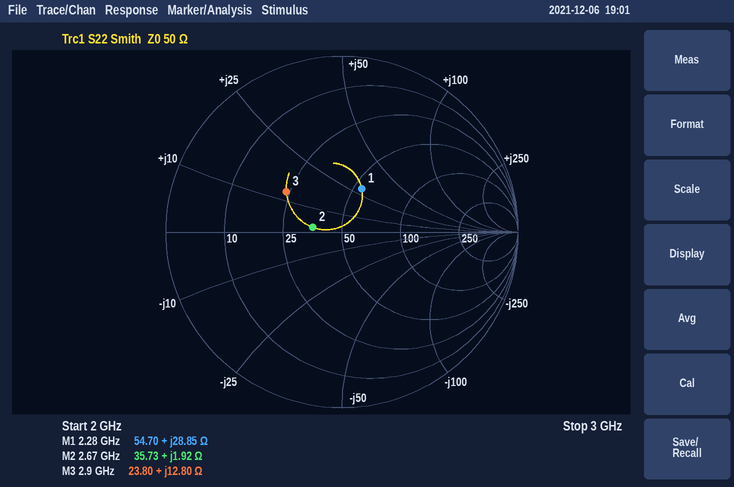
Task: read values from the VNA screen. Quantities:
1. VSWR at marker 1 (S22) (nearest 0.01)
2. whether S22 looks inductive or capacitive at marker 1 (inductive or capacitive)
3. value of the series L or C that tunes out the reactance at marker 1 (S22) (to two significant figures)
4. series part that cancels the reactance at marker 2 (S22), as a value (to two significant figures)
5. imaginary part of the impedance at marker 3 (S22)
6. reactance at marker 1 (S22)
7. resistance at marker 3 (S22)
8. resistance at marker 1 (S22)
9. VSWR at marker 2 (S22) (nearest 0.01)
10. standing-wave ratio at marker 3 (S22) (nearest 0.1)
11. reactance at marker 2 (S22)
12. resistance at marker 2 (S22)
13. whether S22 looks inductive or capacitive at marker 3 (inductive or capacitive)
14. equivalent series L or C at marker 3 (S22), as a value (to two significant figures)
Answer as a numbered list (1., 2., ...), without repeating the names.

1. 1.74
2. inductive
3. 2.4 pF
4. 31 pF
5. +12.80 Ω
6. +28.85 Ω
7. 23.80 Ω
8. 54.70 Ω
9. 1.40
10. 2.3
11. +1.92 Ω
12. 35.73 Ω
13. inductive
14. 700 pH
